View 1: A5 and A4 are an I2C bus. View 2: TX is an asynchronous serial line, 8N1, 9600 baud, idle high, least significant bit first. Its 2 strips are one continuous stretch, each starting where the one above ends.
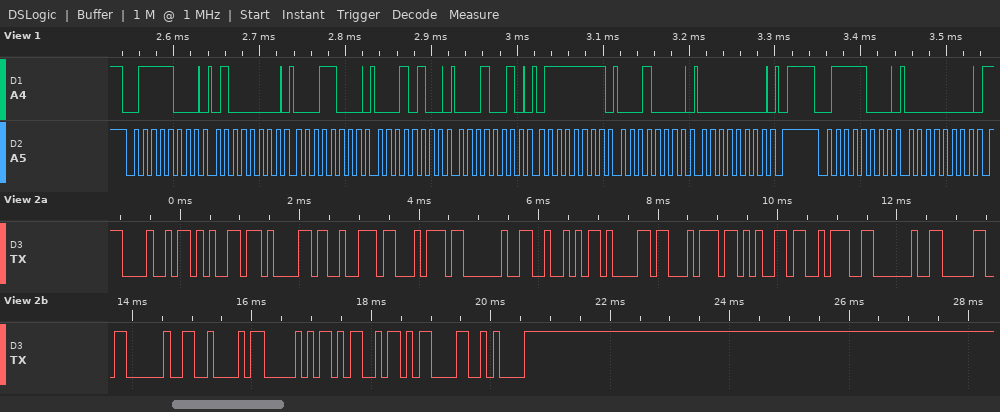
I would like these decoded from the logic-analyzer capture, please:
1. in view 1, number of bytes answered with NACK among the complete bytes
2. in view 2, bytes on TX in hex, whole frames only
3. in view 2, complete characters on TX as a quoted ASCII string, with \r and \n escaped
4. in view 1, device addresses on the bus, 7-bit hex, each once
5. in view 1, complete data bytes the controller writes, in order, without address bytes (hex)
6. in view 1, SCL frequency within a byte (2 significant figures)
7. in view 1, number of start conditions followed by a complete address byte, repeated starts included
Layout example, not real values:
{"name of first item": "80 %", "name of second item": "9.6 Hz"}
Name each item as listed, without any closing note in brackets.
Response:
{"in view 1, number of bytes answered with NACK among the complete bytes": "0", "in view 2, bytes on TX in hex, whole frames only": "48 65 61 72 74 20 52 61 74 65 3A 20 30 20 42 50 4D 0D 0A", "in view 2, complete characters on TX as a quoted ASCII string, with \\r and \\n escaped": "\"Heart Rate: 0 BPM\\r\\n\"", "in view 1, device addresses on the bus, 7-bit hex, each once": "0x3C", "in view 1, complete data bytes the controller writes, in order, without address bytes": "40 18 14 12 7F 10 00 00", "in view 1, SCL frequency within a byte": "100 kHz", "in view 1, number of start conditions followed by a complete address byte, repeated starts included": "2"}
